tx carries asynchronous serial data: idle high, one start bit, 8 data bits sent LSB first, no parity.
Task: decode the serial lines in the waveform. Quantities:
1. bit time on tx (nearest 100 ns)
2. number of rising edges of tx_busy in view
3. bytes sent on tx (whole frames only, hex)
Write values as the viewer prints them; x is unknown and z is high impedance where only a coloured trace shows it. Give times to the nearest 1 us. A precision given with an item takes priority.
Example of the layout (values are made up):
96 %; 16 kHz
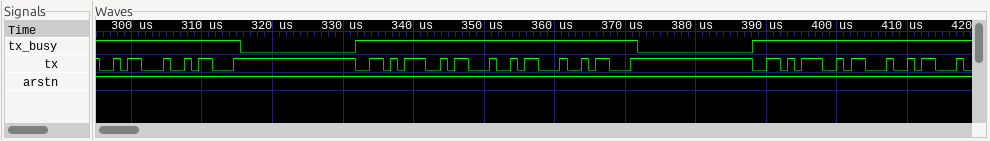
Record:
1000 ns; 2; 1A, 1A, D6, 1A, 1A, 1A, D6, 1A, 1A
